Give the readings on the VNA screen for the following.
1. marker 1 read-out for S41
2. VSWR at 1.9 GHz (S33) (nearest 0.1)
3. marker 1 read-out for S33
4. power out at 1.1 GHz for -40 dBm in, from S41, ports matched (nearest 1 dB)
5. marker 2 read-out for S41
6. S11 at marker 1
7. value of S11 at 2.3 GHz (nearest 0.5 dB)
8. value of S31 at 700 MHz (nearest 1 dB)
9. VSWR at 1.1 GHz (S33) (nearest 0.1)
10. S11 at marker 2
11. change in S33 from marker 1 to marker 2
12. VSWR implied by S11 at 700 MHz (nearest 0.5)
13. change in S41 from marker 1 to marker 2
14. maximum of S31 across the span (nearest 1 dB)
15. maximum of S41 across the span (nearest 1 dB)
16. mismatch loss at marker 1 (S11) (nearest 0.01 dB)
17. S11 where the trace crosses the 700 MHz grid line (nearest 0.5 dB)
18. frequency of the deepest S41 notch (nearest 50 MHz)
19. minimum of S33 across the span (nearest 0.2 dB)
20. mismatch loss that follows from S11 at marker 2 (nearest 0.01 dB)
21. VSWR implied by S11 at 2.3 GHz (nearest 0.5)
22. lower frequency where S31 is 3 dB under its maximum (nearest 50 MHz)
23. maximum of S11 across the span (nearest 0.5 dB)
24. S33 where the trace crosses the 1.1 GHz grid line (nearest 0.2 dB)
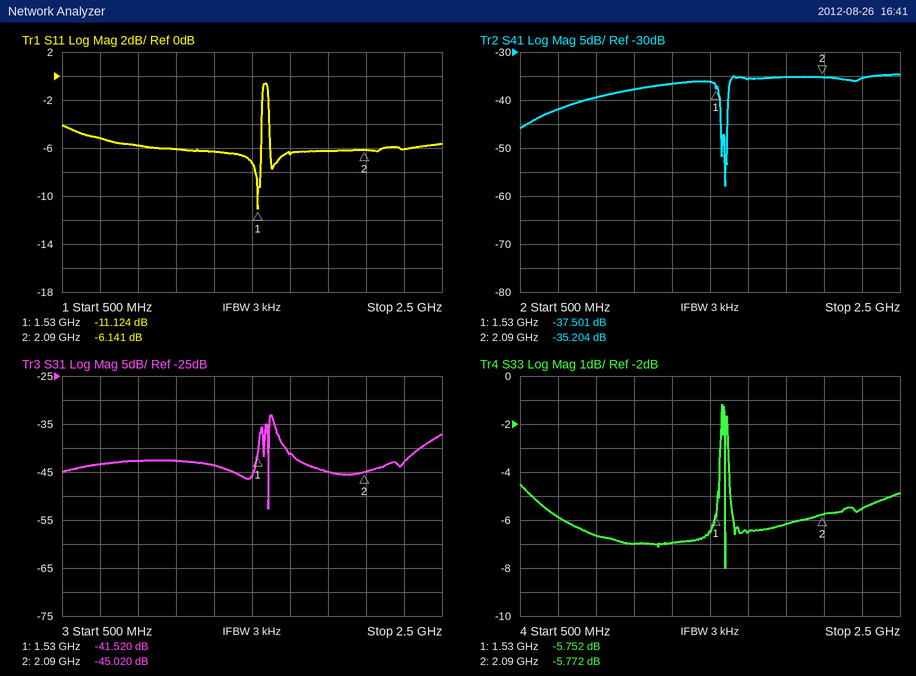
-37.501 dB
2.9
-5.752 dB
-78 dBm
-35.204 dB
-11.124 dB
-6.0 dB
-43 dB
2.6
-6.141 dB
-0.020 dB
3.5
2.297 dB
-33 dB
-35 dB
0.35 dB
-5.0 dB
1.60 GHz
-8.0 dB
1.21 dB
3.0
1.60 GHz
-0.5 dB
-7.0 dB
